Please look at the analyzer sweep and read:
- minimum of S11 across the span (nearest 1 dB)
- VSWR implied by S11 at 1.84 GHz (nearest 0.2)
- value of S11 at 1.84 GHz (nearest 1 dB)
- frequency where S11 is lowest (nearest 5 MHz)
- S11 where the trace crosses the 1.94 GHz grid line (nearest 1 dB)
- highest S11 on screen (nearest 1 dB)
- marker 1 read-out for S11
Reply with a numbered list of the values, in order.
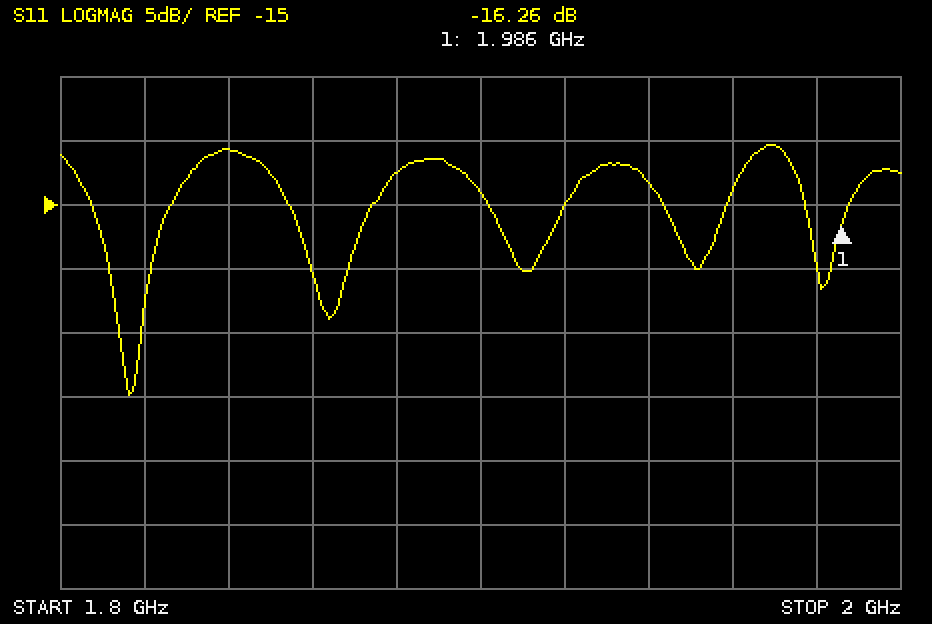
1. -30 dB
2. 1.8
3. -11 dB
4. 1.815 GHz
5. -13 dB
6. -10 dB
7. -16.26 dB
